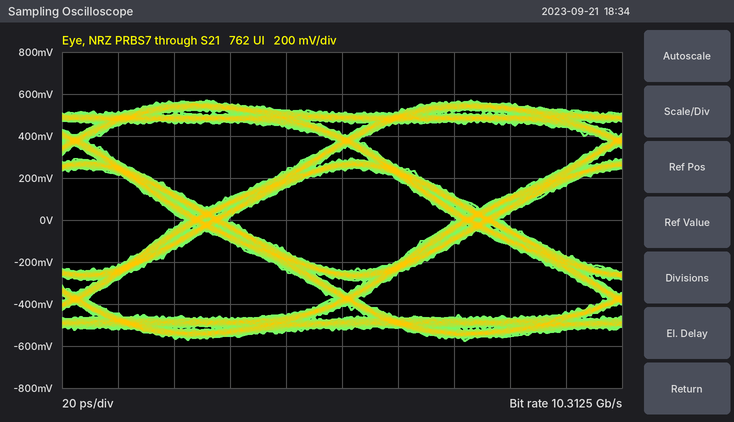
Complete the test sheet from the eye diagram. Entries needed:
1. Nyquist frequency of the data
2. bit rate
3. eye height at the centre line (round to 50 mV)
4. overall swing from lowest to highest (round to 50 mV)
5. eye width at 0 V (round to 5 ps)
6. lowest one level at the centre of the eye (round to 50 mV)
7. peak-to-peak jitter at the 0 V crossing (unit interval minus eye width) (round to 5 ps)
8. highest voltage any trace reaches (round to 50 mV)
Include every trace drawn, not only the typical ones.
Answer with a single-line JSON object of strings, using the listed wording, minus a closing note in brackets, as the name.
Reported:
{"Nyquist frequency of the data": "5.15625 GHz", "bit rate": "10.3125 Gb/s", "eye height at the centre line": "500 mV", "overall swing from lowest to highest": "1.15 V", "eye width at 0 V": "80 ps", "lowest one level at the centre of the eye": "250 mV", "peak-to-peak jitter at the 0 V crossing (unit interval minus eye width)": "15 ps", "highest voltage any trace reaches": "550 mV"}
